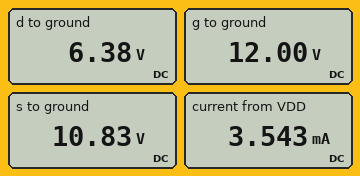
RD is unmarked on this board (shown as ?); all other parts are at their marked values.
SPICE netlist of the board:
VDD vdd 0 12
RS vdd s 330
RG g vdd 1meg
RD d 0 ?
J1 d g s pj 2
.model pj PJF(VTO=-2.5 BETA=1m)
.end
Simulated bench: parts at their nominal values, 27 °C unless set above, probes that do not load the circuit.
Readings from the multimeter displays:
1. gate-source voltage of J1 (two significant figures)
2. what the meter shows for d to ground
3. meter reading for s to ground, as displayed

1.2 V
6.38 V
10.83 V
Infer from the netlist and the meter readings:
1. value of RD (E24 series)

1.8 kΩ
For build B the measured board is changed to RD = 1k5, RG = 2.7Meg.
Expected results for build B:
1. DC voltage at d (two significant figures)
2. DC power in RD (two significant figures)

5.3 V
19 mW
